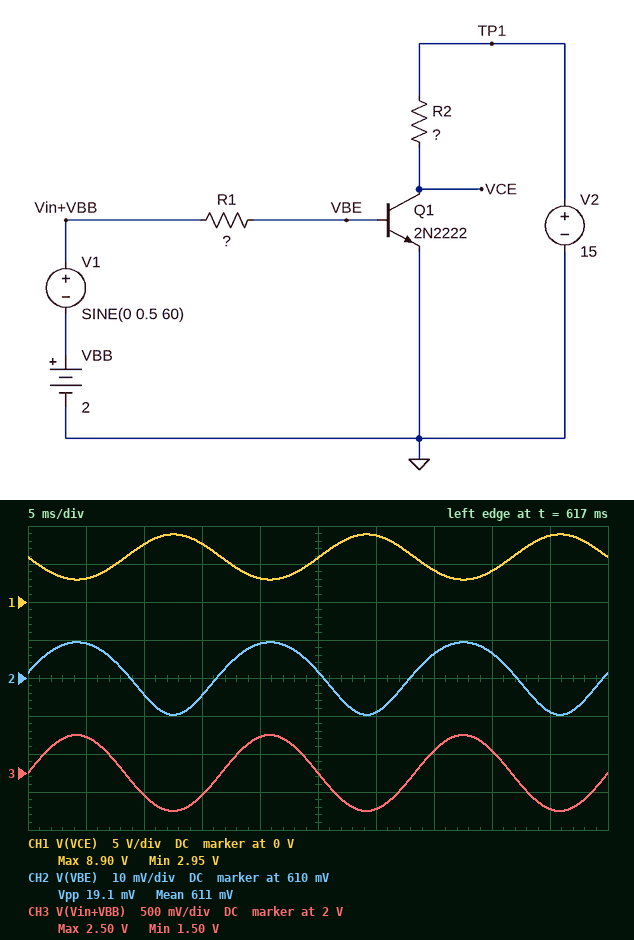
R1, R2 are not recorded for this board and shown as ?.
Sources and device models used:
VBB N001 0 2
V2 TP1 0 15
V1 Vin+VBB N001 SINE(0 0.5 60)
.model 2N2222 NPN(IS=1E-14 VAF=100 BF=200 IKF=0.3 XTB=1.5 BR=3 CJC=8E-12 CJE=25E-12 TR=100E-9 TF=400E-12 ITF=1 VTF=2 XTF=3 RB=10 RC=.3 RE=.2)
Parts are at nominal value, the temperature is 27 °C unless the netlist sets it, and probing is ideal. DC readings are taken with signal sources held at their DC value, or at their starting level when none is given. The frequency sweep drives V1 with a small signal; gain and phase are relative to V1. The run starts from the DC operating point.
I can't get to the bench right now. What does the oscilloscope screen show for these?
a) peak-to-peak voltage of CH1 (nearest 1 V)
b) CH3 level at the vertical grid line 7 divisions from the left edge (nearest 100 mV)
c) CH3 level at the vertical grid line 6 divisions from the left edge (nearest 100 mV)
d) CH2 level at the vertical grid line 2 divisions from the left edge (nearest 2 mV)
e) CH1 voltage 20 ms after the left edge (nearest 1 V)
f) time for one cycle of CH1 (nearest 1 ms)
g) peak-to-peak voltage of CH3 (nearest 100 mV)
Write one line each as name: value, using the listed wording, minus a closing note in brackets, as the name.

peak-to-peak voltage of CH1: 6 V
CH3 level at the vertical grid line 7 divisions from the left edge: 2.3 V
CH3 level at the vertical grid line 6 divisions from the left edge: 1.5 V
CH2 level at the vertical grid line 2 divisions from the left edge: 606 mV
CH1 voltage 20 ms after the left edge: 3 V
time for one cycle of CH1: 17 ms
peak-to-peak voltage of CH3: 1.0 V
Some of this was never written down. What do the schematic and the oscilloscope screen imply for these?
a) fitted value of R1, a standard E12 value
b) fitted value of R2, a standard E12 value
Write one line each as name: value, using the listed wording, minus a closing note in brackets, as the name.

fitted value of R1, a standard E12 value: 1.5 MΩ
fitted value of R2, a standard E12 value: 47 kΩ
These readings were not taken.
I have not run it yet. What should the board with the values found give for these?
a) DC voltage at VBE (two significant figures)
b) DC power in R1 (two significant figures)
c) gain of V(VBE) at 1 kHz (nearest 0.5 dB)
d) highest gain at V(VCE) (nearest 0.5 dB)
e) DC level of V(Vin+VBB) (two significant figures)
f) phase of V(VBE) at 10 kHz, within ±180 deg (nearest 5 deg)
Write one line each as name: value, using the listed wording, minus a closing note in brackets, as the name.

DC voltage at VBE: 610 mV
DC power in R1: 1.3 µW
gain of V(VBE) at 1 kHz: -35.0 dB
highest gain at V(VCE): 15.5 dB
DC level of V(Vin+VBB): 2.0 V
phase of V(VBE) at 10 kHz, within ±180 deg: -65 deg
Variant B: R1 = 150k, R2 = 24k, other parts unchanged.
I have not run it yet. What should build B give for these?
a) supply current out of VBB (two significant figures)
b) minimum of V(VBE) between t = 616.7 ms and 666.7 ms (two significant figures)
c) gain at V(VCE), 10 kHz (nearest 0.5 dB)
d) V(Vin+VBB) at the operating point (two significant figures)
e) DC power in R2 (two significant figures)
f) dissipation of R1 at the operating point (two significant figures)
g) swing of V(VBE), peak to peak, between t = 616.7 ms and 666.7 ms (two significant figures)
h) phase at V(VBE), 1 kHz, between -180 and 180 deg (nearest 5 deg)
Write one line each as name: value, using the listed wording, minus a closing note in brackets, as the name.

supply current out of VBB: 9.0 µA
minimum of V(VBE) between t = 616.7 ms and 666.7 ms: 640 mV
gain at V(VCE), 10 kHz: -31.0 dB
V(Vin+VBB) at the operating point: 2.0 V
DC power in R2: 9.3 mW
dissipation of R1 at the operating point: 12 µW
swing of V(VBE), peak to peak, between t = 616.7 ms and 666.7 ms: 1.2 mV
phase at V(VBE), 1 kHz, between -180 and 180 deg: 0 deg
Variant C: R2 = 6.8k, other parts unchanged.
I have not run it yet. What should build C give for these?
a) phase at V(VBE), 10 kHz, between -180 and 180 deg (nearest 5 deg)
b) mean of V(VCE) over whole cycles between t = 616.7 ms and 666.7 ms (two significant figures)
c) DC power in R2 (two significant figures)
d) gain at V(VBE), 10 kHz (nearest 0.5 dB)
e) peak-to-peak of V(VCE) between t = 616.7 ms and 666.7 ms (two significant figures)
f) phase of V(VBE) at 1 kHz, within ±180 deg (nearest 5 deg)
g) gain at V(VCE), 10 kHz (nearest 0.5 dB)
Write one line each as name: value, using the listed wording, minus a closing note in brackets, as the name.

phase at V(VBE), 10 kHz, between -180 and 180 deg: -20 deg
mean of V(VCE) over whole cycles between t = 616.7 ms and 666.7 ms: 14 V
DC power in R2: 300 µW
gain at V(VBE), 10 kHz: -35.5 dB
peak-to-peak of V(VCE) between t = 616.7 ms and 666.7 ms: 990 mV
phase of V(VBE) at 1 kHz, within ±180 deg: 0 deg
gain at V(VCE), 10 kHz: -0.5 dB
